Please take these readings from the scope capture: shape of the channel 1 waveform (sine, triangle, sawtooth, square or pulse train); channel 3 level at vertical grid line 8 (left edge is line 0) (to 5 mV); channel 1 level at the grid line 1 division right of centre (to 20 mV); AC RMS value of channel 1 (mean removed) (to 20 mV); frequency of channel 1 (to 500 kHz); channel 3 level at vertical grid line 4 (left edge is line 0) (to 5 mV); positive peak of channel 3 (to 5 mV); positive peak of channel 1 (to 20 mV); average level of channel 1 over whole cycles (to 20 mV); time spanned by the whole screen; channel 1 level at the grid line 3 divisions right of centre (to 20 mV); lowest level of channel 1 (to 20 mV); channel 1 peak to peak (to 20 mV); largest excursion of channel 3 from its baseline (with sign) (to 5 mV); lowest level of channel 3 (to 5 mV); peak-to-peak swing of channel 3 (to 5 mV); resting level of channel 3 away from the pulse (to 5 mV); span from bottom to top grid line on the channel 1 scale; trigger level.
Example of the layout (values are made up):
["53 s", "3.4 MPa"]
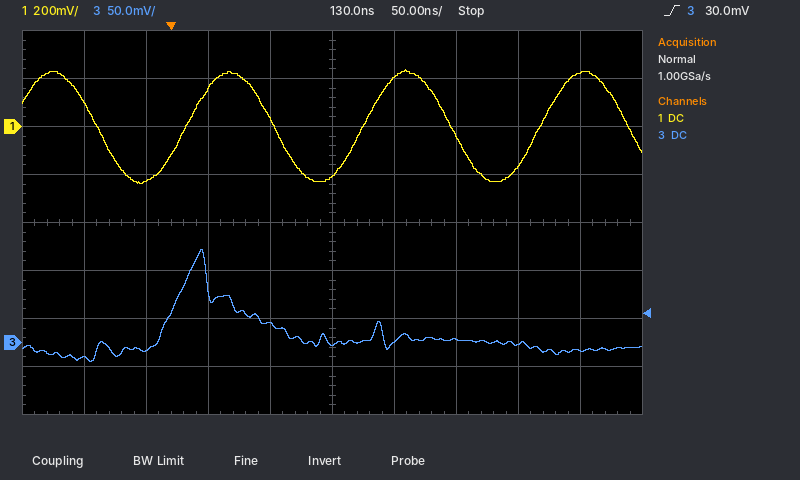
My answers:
["sine", "0 mV", "200 mV", "160 mV", "7.0 MHz", "20 mV", "95 mV", "240 mV", "0 mV", "500 ns", "-160 mV", "-240 mV", "480 mV", "+95 mV", "-20 mV", "115 mV", "0 mV", "1.6 V", "30.0 mV"]
